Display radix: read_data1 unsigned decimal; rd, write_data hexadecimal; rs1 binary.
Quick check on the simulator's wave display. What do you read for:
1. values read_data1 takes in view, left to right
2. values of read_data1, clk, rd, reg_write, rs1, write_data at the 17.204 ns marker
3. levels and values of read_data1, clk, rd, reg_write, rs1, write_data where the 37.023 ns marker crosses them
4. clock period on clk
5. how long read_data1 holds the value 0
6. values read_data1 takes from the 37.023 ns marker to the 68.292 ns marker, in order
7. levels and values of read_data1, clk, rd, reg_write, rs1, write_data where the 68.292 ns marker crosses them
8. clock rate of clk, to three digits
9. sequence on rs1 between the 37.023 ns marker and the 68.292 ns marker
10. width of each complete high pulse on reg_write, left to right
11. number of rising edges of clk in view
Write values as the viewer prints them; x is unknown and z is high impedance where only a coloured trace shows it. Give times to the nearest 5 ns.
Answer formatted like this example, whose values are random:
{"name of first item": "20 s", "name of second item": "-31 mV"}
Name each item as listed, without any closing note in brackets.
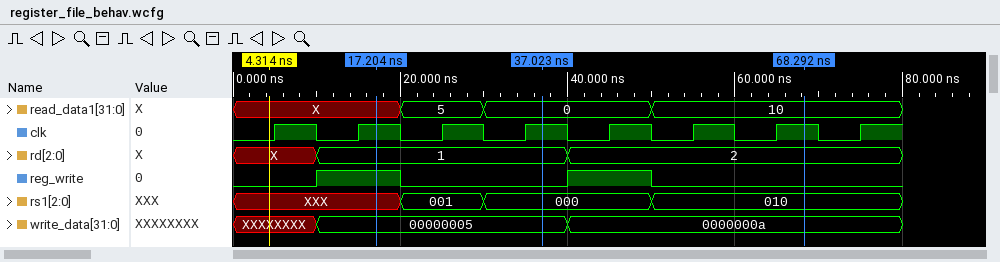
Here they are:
{"values read_data1 takes in view, left to right": "X, 5, 0, 10", "values of read_data1, clk, rd, reg_write, rs1, write_data at the 17.204 ns marker": "read_data1=X, clk=1, rd=1, reg_write=1, rs1=XXX, write_data=00000005", "levels and values of read_data1, clk, rd, reg_write, rs1, write_data where the 37.023 ns marker crosses them": "read_data1=0, clk=1, rd=1, reg_write=0, rs1=000, write_data=00000005", "clock period on clk": "10 ns", "how long read_data1 holds the value 0": "20 ns", "values read_data1 takes from the 37.023 ns marker to the 68.292 ns marker, in order": "0, 10", "levels and values of read_data1, clk, rd, reg_write, rs1, write_data where the 68.292 ns marker crosses them": "read_data1=10, clk=1, rd=2, reg_write=0, rs1=010, write_data=0000000a", "clock rate of clk, to three digits": "100 MHz", "sequence on rs1 between the 37.023 ns marker and the 68.292 ns marker": "000, 010", "width of each complete high pulse on reg_write, left to right": "10 ns, 10 ns", "number of rising edges of clk in view": "8"}
